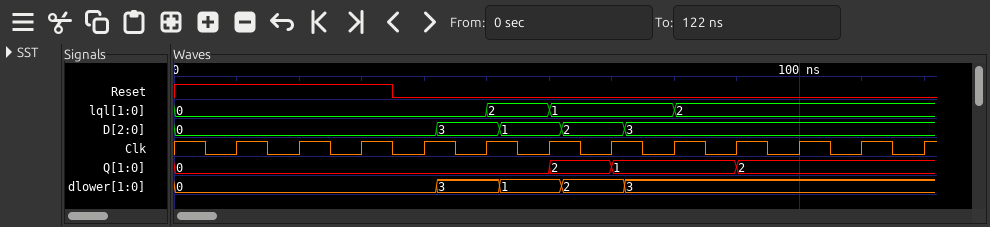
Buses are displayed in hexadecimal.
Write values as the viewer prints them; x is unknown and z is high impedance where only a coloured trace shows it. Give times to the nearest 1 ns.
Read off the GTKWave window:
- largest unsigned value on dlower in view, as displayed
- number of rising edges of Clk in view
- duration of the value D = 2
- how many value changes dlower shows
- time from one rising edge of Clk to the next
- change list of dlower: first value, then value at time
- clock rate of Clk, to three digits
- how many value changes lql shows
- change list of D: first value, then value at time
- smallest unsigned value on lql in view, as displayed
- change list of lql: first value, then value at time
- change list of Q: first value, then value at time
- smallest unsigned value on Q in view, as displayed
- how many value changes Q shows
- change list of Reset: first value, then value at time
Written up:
3
12
10 ns
4
10 ns
0, 3 at 42 ns, 1 at 52 ns, 2 at 62 ns, 3 at 72 ns
100 MHz
3
0, 3 at 42 ns, 1 at 52 ns, 2 at 62 ns, 3 at 72 ns
0
0, 2 at 50 ns, 1 at 60 ns, 2 at 80 ns
0, 2 at 60 ns, 1 at 70 ns, 2 at 90 ns
0
3
1, 0 at 35 ns
